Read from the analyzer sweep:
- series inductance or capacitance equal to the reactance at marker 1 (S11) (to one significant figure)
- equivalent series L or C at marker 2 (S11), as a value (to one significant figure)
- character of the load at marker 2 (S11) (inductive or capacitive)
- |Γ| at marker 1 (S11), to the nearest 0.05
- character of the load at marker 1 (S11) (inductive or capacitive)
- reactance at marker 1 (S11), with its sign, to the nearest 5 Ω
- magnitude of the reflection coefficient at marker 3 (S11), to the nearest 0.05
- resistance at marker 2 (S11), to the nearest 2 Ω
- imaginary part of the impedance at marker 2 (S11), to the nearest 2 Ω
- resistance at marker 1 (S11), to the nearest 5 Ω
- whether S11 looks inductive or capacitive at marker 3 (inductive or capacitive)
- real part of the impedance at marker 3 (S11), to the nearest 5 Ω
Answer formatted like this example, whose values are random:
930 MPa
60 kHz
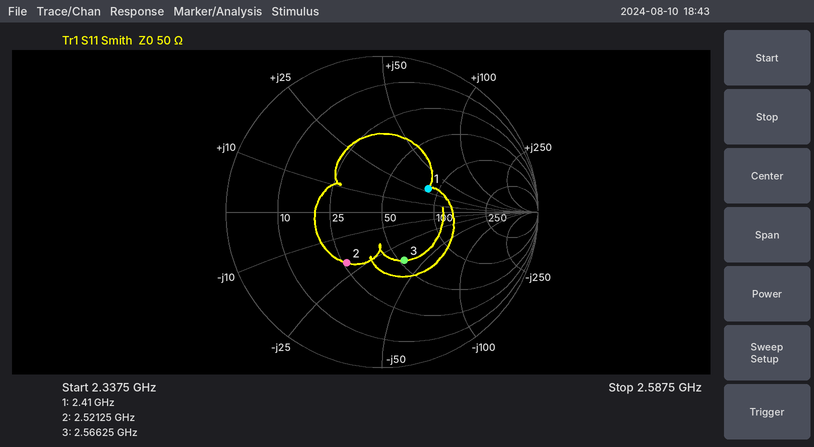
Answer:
2 nH
3 pF
capacitive
0.35
inductive
+30 Ω
0.35
26 Ω
-20 Ω
85 Ω
capacitive
55 Ω
